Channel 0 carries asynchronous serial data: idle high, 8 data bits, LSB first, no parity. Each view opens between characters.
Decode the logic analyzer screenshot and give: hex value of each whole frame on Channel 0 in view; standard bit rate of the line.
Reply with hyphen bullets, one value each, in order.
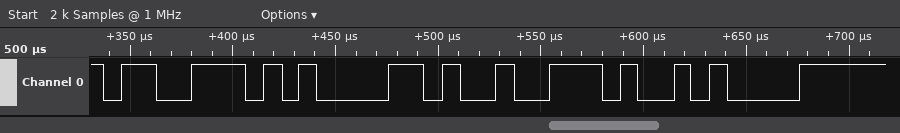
- 73, 61, 72, 0A
- 115200 baud
